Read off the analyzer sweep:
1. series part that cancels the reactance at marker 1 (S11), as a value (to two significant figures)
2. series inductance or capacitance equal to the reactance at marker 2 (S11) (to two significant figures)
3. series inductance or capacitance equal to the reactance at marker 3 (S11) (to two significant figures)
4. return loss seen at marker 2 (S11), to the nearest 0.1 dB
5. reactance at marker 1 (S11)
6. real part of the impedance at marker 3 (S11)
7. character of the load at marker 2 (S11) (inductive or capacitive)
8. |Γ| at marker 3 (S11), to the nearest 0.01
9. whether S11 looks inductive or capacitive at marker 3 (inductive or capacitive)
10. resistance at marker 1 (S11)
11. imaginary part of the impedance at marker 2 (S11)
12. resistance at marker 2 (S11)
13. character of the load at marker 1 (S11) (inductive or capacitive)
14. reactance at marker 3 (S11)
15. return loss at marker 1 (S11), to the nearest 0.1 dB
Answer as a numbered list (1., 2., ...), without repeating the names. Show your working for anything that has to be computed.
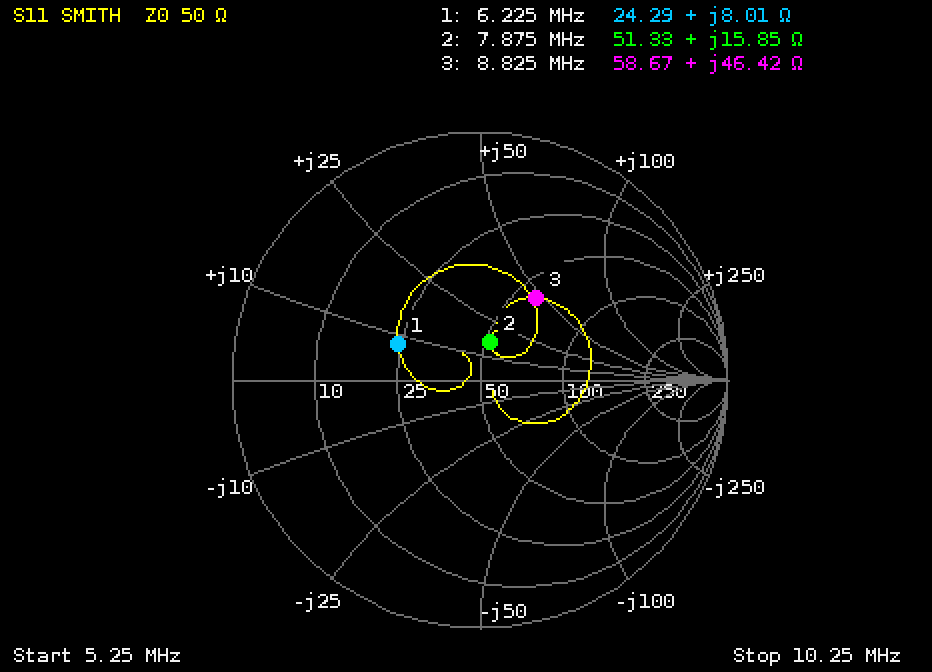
1. C = 1/(2π × 6.225 MHz × 8.01 Ω) ≈ 3.2 nF
2. L = 15.85 Ω/(2π × 7.875 MHz) ≈ 320 nH
3. L = 46.42 Ω/(2π × 8.825 MHz) ≈ 837 nH, so 840 nH to two significant figures
4. 16.2 dB
5. +8.01 Ω
6. 58.67 Ω
7. inductive
8. 0.40
9. inductive
10. 24.29 Ω
11. +15.85 Ω
12. 51.33 Ω
13. inductive
14. +46.42 Ω
15. 8.9 dB
